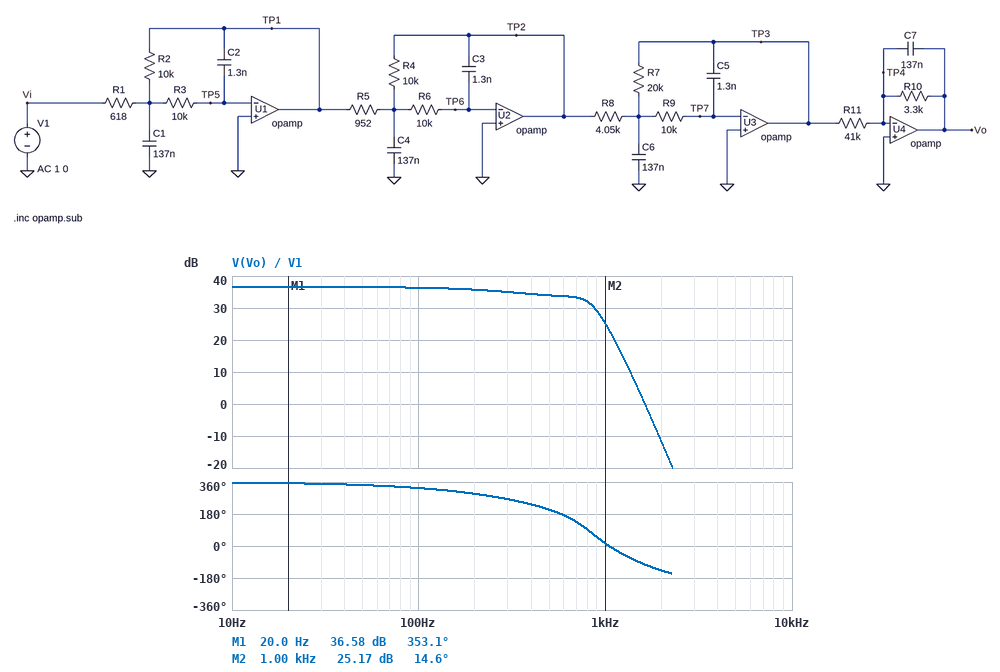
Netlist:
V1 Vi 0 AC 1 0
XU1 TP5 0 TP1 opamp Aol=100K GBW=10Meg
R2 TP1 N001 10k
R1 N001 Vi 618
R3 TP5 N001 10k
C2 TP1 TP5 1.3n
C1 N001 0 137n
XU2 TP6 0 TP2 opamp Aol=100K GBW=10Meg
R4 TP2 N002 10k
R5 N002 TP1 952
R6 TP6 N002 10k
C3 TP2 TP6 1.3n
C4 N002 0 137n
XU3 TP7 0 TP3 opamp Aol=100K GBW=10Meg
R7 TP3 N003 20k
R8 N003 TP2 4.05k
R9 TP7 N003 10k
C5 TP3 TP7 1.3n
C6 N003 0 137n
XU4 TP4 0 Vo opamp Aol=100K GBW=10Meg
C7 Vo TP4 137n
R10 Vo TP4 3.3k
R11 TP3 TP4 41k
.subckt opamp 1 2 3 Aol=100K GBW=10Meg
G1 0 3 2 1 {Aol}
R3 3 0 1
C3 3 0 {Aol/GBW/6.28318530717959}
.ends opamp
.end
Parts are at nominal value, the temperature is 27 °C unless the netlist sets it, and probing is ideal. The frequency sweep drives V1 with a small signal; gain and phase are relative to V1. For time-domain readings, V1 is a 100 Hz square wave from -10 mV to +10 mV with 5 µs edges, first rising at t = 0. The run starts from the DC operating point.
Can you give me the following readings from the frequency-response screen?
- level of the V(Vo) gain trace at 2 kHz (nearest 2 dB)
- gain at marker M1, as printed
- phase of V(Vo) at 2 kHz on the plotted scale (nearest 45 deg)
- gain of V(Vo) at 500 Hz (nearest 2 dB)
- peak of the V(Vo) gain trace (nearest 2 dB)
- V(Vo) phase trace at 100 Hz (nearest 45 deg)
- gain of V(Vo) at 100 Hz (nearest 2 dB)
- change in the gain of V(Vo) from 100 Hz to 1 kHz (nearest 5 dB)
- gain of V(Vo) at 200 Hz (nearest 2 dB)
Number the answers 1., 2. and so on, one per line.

1. -12 dB
2. 36.58 dB
3. -135 deg
4. 34 dB
5. 36 dB
6. 315 deg
7. 36 dB
8. -10 dB
9. 36 dB
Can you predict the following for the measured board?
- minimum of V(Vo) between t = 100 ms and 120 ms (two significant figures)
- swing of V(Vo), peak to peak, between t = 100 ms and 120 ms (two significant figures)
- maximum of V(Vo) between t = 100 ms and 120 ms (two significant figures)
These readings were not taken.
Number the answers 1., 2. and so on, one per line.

1. -690 mV
2. 1.4 V
3. 690 mV
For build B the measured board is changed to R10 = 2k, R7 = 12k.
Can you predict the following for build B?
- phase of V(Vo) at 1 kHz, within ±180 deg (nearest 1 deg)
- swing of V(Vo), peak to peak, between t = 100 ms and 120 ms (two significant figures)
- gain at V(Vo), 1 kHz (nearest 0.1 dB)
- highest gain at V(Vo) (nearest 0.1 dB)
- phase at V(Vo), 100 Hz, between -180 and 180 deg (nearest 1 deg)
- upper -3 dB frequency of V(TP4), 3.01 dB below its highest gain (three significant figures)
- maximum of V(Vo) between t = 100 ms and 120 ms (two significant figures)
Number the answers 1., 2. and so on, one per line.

1. 78 deg
2. 540 mV
3. 24.6 dB
4. 27.8 dB
5. -27 deg
6. 1.16 kHz
7. 270 mV
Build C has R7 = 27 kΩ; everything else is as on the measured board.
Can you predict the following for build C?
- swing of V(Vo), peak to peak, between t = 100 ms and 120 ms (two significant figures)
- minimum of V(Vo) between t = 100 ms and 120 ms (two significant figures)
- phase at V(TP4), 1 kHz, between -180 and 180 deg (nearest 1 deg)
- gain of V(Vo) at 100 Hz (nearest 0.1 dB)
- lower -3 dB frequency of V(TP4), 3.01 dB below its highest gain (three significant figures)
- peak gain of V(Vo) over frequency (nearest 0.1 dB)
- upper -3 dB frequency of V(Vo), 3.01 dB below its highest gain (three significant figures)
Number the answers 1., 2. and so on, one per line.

1. 1.9 V
2. -940 mV
3. -96 deg
4. 39.0 dB
5. 386 Hz
6. 39.2 dB
7. 648 Hz
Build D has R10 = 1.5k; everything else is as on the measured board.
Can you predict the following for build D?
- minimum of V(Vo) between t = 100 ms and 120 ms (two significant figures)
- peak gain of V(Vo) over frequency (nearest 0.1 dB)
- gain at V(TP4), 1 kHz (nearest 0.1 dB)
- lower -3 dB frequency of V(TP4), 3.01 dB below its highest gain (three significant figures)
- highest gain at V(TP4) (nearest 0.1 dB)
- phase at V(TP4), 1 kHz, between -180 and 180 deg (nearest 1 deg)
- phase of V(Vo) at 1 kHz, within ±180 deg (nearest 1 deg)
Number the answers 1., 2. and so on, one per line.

1. -420 mV
2. 30.8 dB
3. -56.3 dB
4. 530 Hz
5. -51.9 dB
6. -63 deg
7. 33 deg
